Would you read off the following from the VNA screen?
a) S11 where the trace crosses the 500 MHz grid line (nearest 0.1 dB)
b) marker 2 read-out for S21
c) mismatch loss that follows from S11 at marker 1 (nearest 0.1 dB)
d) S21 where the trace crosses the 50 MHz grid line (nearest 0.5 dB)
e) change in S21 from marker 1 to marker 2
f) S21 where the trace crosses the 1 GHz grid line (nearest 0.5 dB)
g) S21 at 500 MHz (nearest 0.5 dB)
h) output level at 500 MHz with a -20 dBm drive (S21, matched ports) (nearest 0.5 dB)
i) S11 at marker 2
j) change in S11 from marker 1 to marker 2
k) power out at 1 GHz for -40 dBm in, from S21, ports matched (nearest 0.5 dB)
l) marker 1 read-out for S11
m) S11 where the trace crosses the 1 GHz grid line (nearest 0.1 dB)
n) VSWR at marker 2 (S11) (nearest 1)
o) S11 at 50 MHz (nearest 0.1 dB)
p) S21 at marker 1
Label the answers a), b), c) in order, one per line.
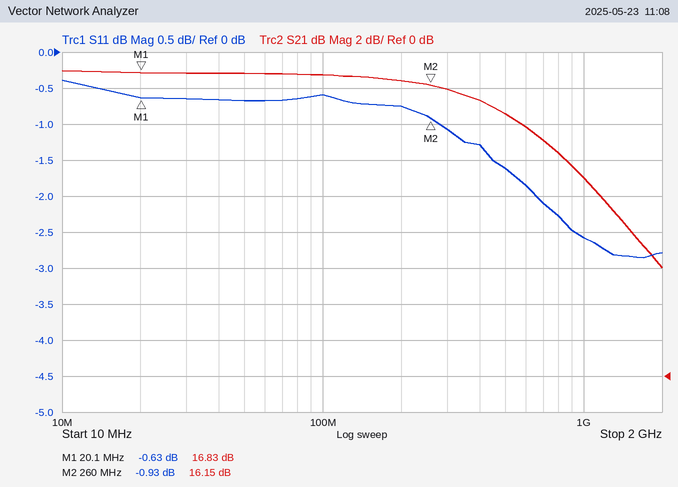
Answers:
a) -1.6 dB
b) 16.15 dB
c) 8.7 dB
d) 17.0 dB
e) -0.68 dB
f) 11.0 dB
g) 14.5 dB
h) -5.5 dBm
i) -0.93 dB
j) -0.30 dB
k) -29.0 dBm
l) -0.63 dB
m) -2.6 dB
n) 19
o) -0.7 dB
p) 16.83 dB
